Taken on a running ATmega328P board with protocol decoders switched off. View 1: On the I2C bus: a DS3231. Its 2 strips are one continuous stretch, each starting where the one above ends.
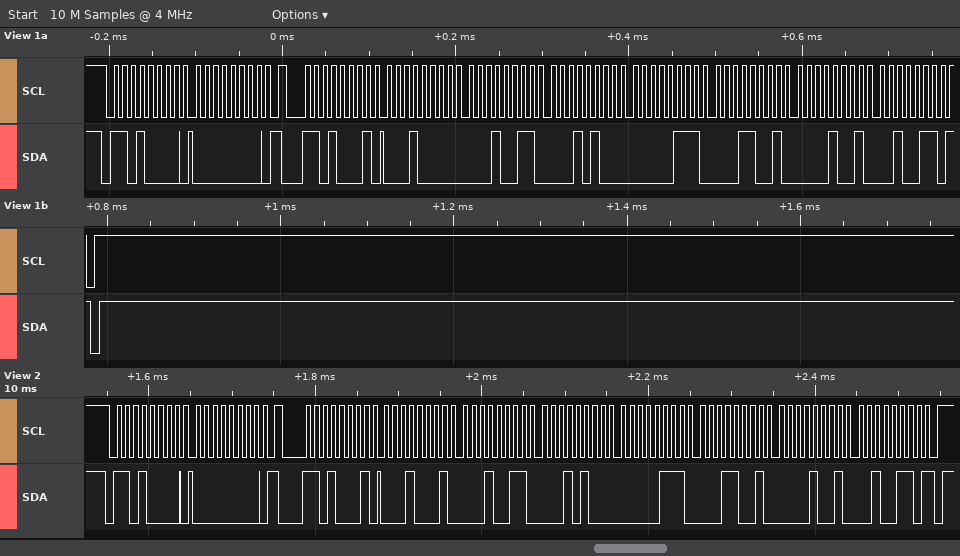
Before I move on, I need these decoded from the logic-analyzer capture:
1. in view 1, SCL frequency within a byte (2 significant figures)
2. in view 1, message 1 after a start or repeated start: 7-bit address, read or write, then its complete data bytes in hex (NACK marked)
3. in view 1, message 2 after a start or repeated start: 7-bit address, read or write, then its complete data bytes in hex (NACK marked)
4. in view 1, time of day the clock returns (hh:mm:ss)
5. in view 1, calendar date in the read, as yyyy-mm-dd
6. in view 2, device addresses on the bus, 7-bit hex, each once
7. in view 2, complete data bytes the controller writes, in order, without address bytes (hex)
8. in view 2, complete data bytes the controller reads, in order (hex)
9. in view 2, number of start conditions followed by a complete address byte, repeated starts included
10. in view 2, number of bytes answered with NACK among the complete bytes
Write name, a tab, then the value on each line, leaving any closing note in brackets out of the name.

in view 1, SCL frequency within a byte	100 kHz
in view 1, message 1 after a start or repeated start: 7-bit address, read or write, then its complete data bytes in hex	0x68 write: 00
in view 1, message 2 after a start or repeated start: 7-bit address, read or write, then its complete data bytes in hex	0x68 read: 10 13 14 07 19 09 26 NACK
in view 1, time of day the clock returns	14:13:10
in view 1, calendar date in the read, as yyyy-mm-dd	2026-09-19
in view 2, device addresses on the bus, 7-bit hex, each once	0x68
in view 2, complete data bytes the controller writes, in order, without address bytes	00
in view 2, complete data bytes the controller reads, in order	11 13 14 07 19 09 26
in view 2, number of start conditions followed by a complete address byte, repeated starts included	2
in view 2, number of bytes answered with NACK among the complete bytes	1
